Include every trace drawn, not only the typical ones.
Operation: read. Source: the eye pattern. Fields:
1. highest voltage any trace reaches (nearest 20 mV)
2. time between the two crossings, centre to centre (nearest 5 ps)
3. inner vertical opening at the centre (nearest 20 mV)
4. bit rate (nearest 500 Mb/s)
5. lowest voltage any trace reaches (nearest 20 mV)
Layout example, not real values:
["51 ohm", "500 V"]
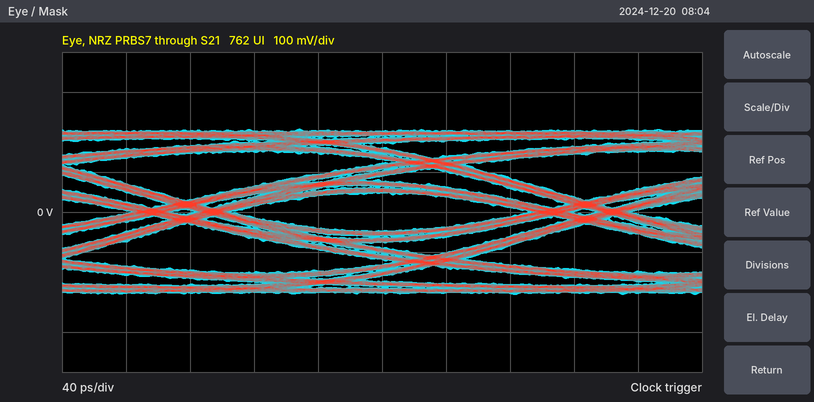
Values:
["200 mV", "250 ps", "100 mV", "4.0 Gb/s", "-200 mV"]
